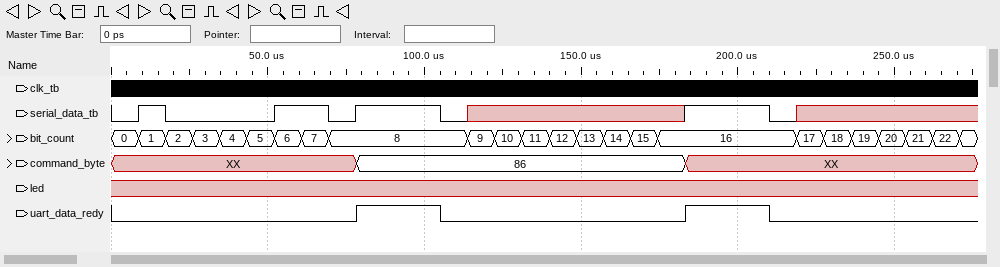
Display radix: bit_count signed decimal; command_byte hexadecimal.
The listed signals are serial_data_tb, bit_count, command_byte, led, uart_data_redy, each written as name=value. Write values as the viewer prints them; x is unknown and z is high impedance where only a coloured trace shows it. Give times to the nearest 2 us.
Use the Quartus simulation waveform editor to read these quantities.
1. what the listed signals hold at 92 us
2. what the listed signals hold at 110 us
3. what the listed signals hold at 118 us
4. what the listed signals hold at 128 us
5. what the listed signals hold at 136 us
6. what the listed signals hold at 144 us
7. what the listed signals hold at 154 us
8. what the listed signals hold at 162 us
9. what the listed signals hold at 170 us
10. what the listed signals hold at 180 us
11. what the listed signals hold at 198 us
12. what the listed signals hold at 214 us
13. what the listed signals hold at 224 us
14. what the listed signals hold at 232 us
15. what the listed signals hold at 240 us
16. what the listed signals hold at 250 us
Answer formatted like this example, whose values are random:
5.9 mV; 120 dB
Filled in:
serial_data_tb=1, bit_count=8, command_byte=86, led=x, uart_data_redy=1; serial_data_tb=0, bit_count=8, command_byte=86, led=x, uart_data_redy=0; serial_data_tb=x, bit_count=9, command_byte=86, led=x, uart_data_redy=0; serial_data_tb=x, bit_count=10, command_byte=86, led=x, uart_data_redy=0; serial_data_tb=x, bit_count=11, command_byte=86, led=x, uart_data_redy=0; serial_data_tb=x, bit_count=12, command_byte=86, led=x, uart_data_redy=0; serial_data_tb=x, bit_count=13, command_byte=86, led=x, uart_data_redy=0; serial_data_tb=x, bit_count=14, command_byte=86, led=x, uart_data_redy=0; serial_data_tb=x, bit_count=15, command_byte=86, led=x, uart_data_redy=0; serial_data_tb=x, bit_count=16, command_byte=86, led=x, uart_data_redy=0; serial_data_tb=1, bit_count=16, command_byte=XX, led=x, uart_data_redy=1; serial_data_tb=0, bit_count=16, command_byte=XX, led=x, uart_data_redy=0; serial_data_tb=x, bit_count=17, command_byte=XX, led=x, uart_data_redy=0; serial_data_tb=x, bit_count=18, command_byte=XX, led=x, uart_data_redy=0; serial_data_tb=x, bit_count=19, command_byte=XX, led=x, uart_data_redy=0; serial_data_tb=x, bit_count=20, command_byte=XX, led=x, uart_data_redy=0
